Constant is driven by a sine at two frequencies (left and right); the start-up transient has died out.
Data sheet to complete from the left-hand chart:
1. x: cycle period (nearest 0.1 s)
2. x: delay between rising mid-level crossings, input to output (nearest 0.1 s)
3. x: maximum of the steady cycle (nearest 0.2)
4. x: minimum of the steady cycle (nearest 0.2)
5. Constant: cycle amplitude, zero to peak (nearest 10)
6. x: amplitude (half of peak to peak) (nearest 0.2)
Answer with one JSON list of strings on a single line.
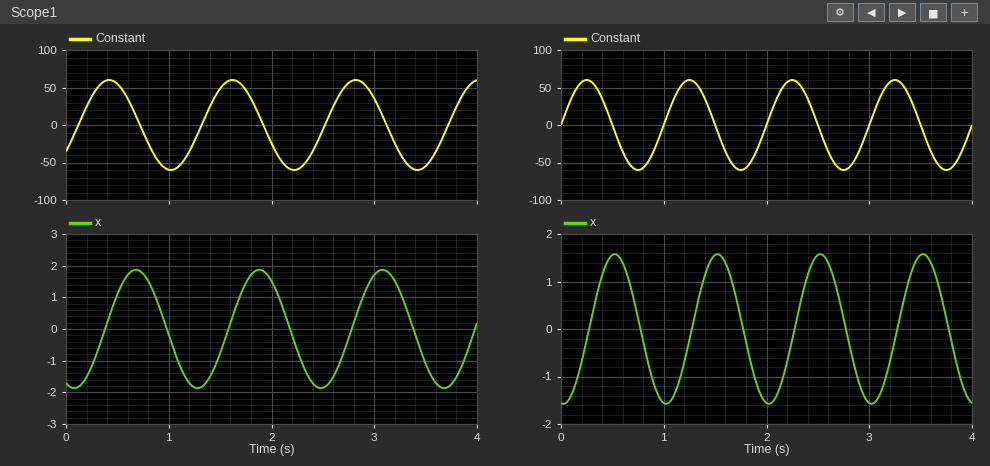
["1.2 s", "0.3 s", "1.8", "-1.8", "60", "1.8"]
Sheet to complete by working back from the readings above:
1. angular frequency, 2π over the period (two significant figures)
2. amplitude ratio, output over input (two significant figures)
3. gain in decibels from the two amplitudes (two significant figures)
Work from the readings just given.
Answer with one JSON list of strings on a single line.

["5.2 rad/s", "0.030", "-30 dB"]
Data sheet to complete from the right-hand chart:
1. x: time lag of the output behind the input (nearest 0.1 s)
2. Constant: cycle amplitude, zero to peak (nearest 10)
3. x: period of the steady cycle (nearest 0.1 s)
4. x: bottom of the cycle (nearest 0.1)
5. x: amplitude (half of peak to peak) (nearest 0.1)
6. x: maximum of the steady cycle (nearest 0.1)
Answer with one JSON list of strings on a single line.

["0.3 s", "60", "1.0 s", "-1.6", "1.6", "1.6"]
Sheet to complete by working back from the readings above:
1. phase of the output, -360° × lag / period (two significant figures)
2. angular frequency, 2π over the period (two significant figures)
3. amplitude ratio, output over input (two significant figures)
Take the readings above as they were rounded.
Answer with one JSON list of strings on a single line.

["-110°", "6.3 rad/s", "0.027"]
